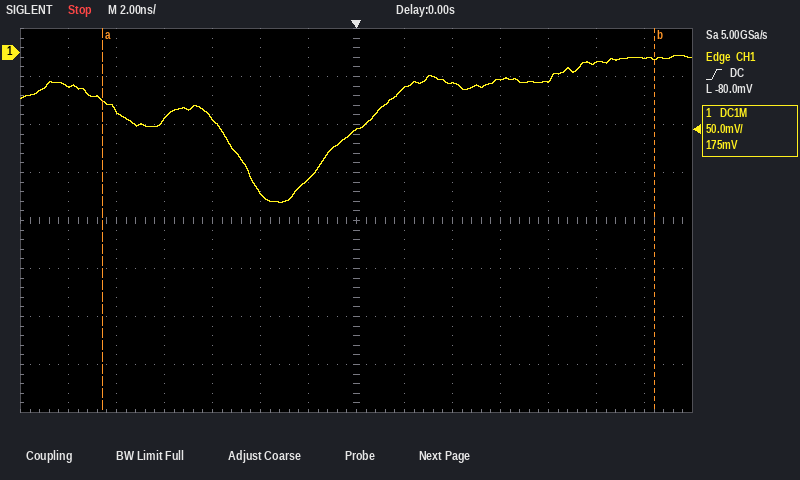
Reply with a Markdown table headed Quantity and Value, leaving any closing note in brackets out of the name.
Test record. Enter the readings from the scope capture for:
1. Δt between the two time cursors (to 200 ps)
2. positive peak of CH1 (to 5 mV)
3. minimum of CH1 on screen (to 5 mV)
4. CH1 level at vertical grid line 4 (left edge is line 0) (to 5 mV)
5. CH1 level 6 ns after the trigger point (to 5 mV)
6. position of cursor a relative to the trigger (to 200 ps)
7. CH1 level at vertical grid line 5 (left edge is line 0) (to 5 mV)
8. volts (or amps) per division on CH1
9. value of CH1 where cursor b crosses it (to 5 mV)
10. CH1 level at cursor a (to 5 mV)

| Quantity | Value |
|---|---|
| Δt between the two time cursors | 23.0 ns |
| positive peak of CH1 | -5 mV |
| minimum of CH1 on screen | -155 mV |
| CH1 level at vertical grid line 4 (left edge is line 0) | -70 mV |
| CH1 level 6 ns after the trigger point | -30 mV |
| position of cursor a relative to the trigger | -10.6 ns |
| CH1 level at vertical grid line 5 (left edge is line 0) | -145 mV |
| volts (or amps) per division on CH1 | 50 mV |
| value of CH1 where cursor b crosses it | -5 mV |
| CH1 level at cursor a | -50 mV |
